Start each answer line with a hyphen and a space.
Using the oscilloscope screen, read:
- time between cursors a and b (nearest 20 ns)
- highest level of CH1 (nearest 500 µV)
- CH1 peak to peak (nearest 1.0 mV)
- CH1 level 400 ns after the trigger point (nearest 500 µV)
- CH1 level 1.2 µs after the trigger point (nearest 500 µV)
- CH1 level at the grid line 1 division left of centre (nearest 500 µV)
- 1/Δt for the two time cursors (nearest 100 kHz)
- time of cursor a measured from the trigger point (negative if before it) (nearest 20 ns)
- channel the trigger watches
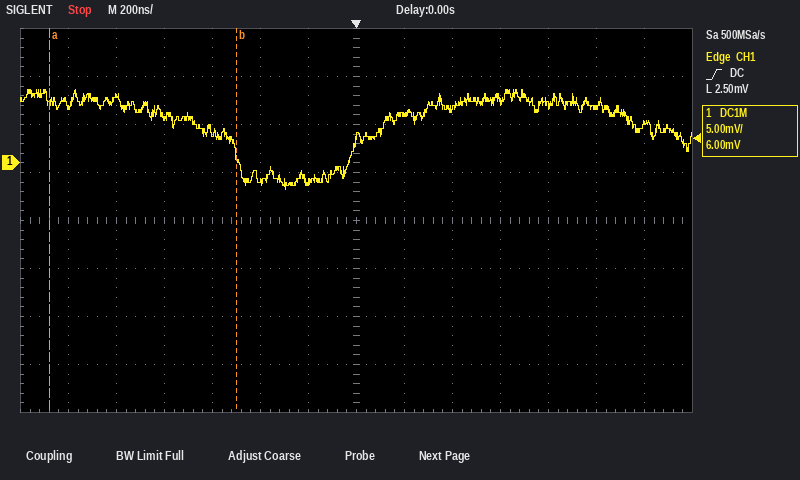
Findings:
- 780 ns
- 7.5 mV
- 10.0 mV
- 5.5 mV
- 4.0 mV
- -2.0 mV
- 1.3 MHz
- -1.28 µs
- CH1
